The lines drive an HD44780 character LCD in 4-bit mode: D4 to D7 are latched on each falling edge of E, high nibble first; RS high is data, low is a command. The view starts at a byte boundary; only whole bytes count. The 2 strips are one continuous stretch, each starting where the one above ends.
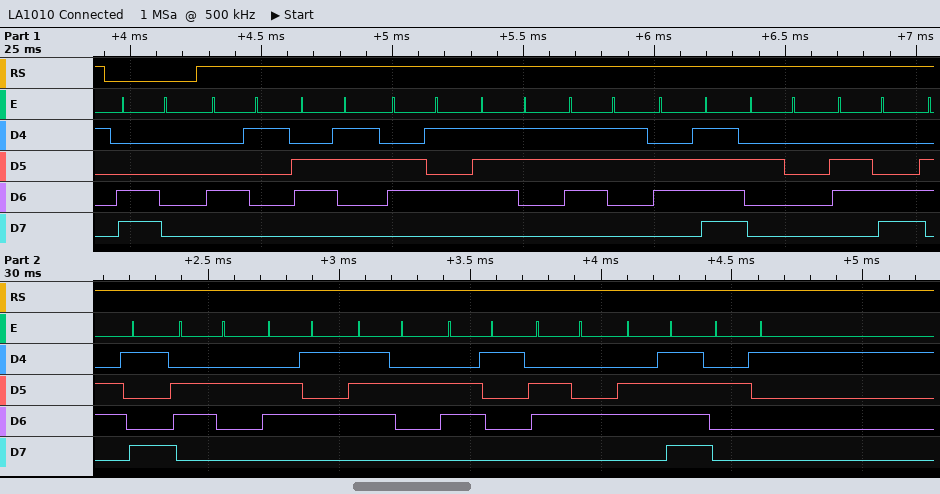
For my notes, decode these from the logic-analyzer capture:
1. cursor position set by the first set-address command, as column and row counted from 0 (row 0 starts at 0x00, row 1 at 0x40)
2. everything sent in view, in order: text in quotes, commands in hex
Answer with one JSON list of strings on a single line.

["column 0, row 1", "0xC0 \"Acesso liberado!\""]
